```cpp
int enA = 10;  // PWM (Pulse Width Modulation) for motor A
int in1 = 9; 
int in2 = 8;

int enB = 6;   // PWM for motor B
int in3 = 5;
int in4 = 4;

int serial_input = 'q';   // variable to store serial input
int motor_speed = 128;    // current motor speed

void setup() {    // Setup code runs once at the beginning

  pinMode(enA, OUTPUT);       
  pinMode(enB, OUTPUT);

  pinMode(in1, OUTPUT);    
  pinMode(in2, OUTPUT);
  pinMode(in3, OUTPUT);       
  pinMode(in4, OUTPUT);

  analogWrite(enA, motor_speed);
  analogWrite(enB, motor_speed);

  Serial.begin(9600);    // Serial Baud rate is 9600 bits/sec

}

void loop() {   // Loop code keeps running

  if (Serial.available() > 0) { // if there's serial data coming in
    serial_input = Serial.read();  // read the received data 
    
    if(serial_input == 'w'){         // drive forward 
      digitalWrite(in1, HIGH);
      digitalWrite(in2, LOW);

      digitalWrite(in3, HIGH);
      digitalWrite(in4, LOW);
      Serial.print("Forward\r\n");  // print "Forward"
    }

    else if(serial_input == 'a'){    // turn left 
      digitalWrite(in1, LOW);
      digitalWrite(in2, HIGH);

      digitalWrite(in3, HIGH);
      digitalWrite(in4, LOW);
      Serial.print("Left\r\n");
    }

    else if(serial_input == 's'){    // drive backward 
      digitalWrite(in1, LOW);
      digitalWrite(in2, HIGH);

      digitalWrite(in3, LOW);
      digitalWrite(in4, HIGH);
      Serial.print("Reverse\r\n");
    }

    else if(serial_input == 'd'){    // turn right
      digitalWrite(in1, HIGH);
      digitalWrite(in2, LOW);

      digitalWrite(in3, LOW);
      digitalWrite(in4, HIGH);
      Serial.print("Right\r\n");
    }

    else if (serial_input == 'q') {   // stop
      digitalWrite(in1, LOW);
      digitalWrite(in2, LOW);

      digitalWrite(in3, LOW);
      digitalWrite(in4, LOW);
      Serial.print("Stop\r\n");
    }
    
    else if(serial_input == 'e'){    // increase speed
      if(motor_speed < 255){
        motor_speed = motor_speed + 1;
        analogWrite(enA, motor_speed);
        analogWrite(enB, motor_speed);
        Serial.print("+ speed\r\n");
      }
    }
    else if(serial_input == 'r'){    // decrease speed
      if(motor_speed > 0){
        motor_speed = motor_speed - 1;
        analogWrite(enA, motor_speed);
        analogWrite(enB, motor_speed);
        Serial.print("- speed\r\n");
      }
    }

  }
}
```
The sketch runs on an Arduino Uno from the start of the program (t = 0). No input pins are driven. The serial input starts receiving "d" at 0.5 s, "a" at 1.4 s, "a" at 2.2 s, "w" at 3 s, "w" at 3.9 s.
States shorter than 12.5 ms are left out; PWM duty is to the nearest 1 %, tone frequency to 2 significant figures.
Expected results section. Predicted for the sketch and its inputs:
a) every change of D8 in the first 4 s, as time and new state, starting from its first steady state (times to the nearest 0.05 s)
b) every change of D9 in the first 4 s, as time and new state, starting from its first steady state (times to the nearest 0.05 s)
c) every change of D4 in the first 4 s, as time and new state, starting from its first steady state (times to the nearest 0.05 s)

0 s low; 1.4 s high; 3 s low
0 s low; 0.5 s high; 1.4 s low; 3 s high
0 s low; 0.5 s high; 1.4 s low
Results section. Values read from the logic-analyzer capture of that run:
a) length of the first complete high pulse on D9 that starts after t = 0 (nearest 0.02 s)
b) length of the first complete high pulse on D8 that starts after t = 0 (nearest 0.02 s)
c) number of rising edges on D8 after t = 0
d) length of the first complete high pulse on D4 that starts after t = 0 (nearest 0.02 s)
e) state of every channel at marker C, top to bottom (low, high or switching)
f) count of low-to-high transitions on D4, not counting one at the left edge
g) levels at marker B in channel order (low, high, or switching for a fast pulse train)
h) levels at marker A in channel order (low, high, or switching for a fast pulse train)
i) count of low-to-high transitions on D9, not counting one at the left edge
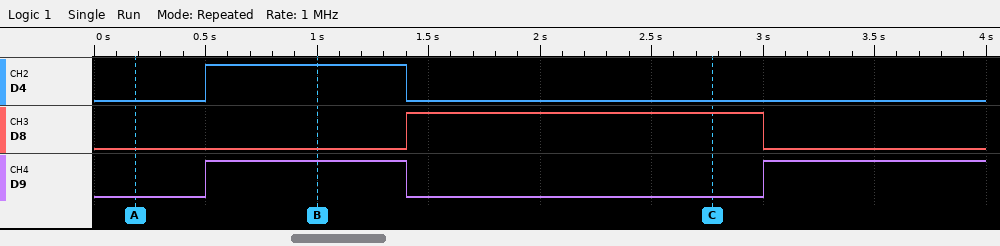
0.90 s
1.60 s
1
0.90 s
D4 low, D8 high, D9 low
1
D4 high, D8 low, D9 high
D4 low, D8 low, D9 low
2
